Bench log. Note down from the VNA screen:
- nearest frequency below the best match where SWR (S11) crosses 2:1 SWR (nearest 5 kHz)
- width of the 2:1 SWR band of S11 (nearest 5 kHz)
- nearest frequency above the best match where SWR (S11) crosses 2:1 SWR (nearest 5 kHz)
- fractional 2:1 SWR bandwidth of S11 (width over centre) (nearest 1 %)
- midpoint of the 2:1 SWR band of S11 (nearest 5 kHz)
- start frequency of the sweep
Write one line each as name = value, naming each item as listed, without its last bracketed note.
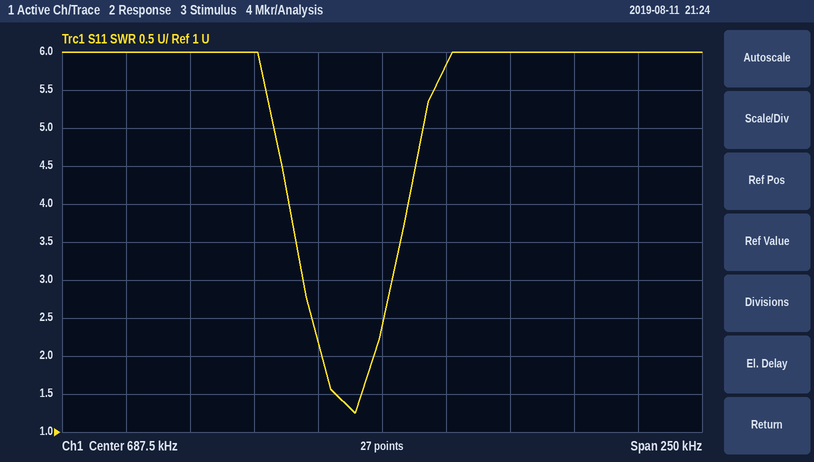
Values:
nearest frequency below the best match where SWR (S11) crosses 2:1 SWR = 665 kHz
width of the 2:1 SWR band of S11 = 20 kHz
nearest frequency above the best match where SWR (S11) crosses 2:1 SWR = 685 kHz
fractional 2:1 SWR bandwidth of S11 (width over centre) = 3 %
midpoint of the 2:1 SWR band of S11 = 675 kHz
start frequency of the sweep = 562.5 kHz
